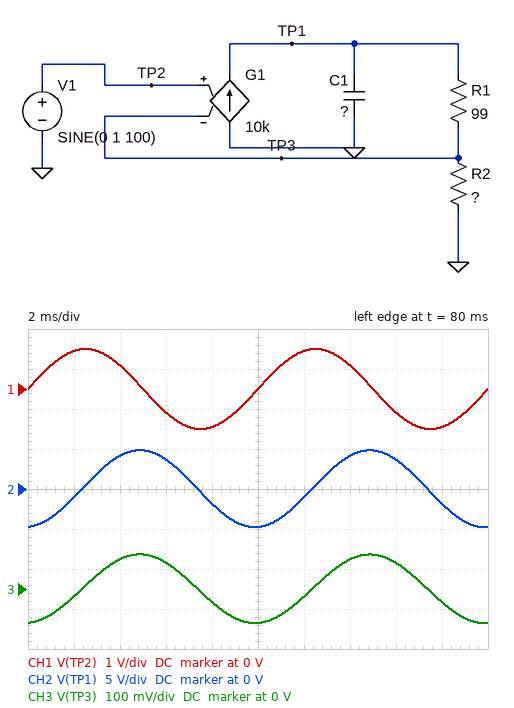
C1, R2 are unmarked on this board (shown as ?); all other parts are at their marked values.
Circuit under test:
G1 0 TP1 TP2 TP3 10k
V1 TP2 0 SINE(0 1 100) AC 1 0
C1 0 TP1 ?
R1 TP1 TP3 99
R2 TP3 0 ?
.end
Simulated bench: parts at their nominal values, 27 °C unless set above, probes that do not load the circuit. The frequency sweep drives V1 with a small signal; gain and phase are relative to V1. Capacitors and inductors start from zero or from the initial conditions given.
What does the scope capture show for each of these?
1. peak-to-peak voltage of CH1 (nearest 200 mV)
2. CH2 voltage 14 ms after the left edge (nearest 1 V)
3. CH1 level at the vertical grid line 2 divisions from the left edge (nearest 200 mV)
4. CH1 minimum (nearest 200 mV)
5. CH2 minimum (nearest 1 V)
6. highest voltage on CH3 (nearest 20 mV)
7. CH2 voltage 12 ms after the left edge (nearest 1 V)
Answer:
2.0 V
4 V
600 mV
-1.0 V
-5 V
80 mV
-1 V
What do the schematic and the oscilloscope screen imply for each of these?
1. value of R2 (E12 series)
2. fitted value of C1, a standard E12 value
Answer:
1.8 Ω
3.3 F
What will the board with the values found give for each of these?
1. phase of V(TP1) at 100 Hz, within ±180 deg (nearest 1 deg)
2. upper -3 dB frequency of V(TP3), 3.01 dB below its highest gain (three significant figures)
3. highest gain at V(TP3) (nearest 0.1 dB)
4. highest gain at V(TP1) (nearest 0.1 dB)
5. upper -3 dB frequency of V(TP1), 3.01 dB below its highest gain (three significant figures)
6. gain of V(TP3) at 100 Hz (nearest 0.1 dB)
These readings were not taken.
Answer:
-85 deg
8.61 Hz
0 dB
35.0 dB
8.61 Hz
-21.3 dB
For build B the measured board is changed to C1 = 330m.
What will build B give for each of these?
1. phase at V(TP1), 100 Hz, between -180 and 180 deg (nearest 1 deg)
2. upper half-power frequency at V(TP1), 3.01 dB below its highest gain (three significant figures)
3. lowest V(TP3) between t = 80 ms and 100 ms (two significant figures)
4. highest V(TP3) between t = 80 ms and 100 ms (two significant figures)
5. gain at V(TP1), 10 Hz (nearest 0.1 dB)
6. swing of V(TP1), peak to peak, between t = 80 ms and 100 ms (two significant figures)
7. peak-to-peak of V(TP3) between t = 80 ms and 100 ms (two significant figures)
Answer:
-49 deg
86.1 Hz
-650 mV
650 mV
34.9 dB
73 V
1.3 V
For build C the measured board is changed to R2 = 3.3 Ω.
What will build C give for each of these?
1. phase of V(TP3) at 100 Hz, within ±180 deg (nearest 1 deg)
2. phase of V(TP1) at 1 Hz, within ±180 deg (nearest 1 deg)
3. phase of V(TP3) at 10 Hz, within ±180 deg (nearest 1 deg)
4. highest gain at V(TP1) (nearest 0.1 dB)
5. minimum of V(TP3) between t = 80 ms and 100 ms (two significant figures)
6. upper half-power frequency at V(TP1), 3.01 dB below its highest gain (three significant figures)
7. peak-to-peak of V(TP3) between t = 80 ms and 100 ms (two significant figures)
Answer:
-81 deg
-4 deg
-33 deg
29.8 dB
-150 mV
15.6 Hz
310 mV
